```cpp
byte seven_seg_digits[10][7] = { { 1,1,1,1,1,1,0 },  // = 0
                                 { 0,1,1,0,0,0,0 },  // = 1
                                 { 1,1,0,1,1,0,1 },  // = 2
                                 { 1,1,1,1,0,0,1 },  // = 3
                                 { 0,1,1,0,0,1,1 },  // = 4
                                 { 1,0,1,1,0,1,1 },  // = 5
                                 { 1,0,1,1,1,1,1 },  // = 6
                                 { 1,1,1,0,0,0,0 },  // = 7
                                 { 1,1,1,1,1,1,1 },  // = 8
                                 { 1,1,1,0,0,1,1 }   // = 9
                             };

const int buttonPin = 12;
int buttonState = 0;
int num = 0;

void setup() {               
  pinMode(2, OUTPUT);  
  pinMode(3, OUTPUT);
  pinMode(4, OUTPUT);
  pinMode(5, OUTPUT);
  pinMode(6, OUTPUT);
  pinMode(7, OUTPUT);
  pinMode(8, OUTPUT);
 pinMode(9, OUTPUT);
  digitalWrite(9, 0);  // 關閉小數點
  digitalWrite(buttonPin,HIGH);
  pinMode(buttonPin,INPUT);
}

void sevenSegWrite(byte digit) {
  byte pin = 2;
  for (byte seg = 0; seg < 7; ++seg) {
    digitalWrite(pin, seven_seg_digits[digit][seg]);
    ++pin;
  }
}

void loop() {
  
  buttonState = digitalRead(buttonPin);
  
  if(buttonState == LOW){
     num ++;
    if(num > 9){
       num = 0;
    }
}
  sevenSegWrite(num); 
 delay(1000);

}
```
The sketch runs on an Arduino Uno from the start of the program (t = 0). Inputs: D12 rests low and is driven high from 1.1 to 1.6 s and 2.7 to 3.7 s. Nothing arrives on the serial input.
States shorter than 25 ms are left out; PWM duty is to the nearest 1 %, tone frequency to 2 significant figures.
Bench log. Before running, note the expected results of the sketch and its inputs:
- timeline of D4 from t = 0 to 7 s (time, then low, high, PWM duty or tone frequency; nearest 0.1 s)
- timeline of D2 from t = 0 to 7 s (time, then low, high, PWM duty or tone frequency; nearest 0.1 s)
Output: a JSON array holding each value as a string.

["0 s high; 1 s low; 2 s high", "0 s low; 1 s high; 4 s low; 5 s high"]
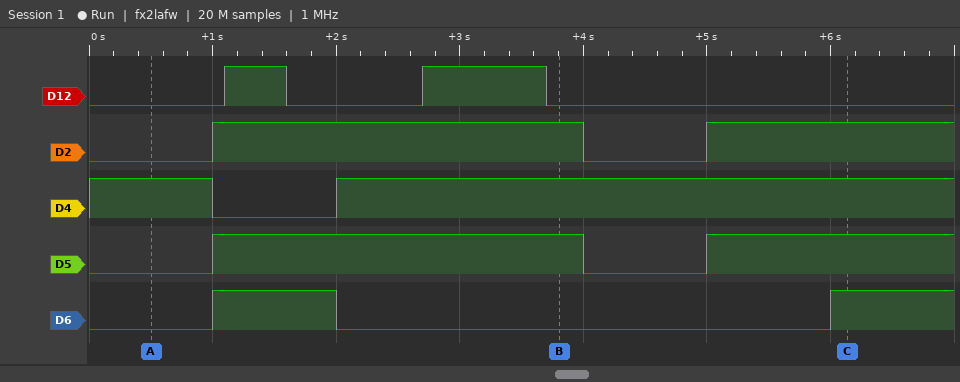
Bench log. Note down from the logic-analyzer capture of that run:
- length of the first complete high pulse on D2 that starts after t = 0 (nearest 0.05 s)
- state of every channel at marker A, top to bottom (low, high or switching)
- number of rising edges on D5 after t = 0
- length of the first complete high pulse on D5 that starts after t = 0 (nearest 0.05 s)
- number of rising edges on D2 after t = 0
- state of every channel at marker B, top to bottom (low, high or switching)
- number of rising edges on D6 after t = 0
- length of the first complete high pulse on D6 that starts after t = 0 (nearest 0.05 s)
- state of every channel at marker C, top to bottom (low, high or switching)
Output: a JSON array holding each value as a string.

["3.00 s", "D12 low, D2 low, D4 high, D5 low, D6 low", "2", "3.00 s", "2", "D12 low, D2 high, D4 high, D5 high, D6 low", "2", "1.00 s", "D12 low, D2 high, D4 high, D5 high, D6 high"]
